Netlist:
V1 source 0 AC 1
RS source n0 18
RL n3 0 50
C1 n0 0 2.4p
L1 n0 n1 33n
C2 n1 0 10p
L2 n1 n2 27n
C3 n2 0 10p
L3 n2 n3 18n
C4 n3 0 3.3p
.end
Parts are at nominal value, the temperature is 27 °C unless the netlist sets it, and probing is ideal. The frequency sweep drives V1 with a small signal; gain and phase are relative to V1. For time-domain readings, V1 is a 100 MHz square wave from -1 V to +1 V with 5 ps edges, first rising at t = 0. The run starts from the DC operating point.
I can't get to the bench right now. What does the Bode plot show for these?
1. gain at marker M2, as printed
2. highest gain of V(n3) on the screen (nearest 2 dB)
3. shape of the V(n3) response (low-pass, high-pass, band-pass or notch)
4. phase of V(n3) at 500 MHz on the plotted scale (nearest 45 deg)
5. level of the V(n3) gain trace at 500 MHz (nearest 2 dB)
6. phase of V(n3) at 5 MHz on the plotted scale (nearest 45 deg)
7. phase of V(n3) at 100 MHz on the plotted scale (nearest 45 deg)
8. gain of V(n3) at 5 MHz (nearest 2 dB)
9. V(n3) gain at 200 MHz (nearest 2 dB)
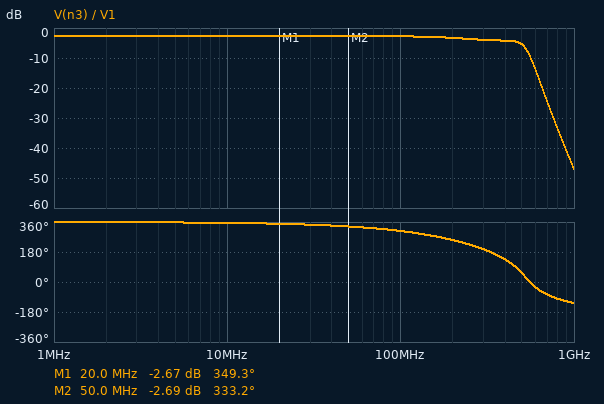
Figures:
-2.69 dB
-2 dB
low-pass
45 deg
-6 dB
360 deg
315 deg
-2 dB
-4 dB
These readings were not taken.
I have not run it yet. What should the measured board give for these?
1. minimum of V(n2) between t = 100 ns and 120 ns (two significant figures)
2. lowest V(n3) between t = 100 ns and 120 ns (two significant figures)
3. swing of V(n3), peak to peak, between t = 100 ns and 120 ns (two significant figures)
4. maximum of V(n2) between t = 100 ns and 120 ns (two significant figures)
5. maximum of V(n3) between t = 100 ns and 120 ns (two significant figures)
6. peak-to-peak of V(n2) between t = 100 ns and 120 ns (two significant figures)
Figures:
-900 mV
-880 mV
1.8 V
900 mV
880 mV
1.8 V
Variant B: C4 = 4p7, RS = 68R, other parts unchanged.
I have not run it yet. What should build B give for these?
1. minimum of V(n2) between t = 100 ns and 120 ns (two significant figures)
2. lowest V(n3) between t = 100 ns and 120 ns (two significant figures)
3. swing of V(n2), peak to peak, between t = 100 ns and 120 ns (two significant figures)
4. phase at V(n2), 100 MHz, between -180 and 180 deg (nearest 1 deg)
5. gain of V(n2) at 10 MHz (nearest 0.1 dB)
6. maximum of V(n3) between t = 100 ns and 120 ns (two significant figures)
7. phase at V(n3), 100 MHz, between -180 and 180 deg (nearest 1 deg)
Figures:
-540 mV
-550 mV
1.1 V
-39 deg
-7.5 dB
550 mV
-52 deg
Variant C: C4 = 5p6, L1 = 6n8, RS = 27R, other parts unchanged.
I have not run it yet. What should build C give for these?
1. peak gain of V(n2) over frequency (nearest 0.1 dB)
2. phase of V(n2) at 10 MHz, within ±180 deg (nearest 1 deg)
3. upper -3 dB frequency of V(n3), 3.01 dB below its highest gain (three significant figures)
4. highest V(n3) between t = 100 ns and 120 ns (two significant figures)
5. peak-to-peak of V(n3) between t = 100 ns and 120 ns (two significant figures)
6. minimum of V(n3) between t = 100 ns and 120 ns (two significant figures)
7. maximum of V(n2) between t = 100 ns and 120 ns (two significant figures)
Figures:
-2.8 dB
-3 deg
614 MHz
820 mV
1.6 V
-820 mV
780 mV
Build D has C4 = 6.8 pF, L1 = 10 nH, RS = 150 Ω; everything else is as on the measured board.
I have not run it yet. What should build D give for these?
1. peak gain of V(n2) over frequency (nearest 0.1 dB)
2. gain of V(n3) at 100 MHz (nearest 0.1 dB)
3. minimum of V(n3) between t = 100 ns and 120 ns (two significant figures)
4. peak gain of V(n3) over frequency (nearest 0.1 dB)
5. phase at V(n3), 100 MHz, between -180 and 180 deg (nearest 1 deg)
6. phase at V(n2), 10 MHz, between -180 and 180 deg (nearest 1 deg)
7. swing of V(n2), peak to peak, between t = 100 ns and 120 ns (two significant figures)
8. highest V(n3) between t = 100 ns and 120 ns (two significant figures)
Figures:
-12.0 dB
-12.4 dB
-300 mV
-11.6 dB
-47 deg
-4 deg
520 mV
300 mV
